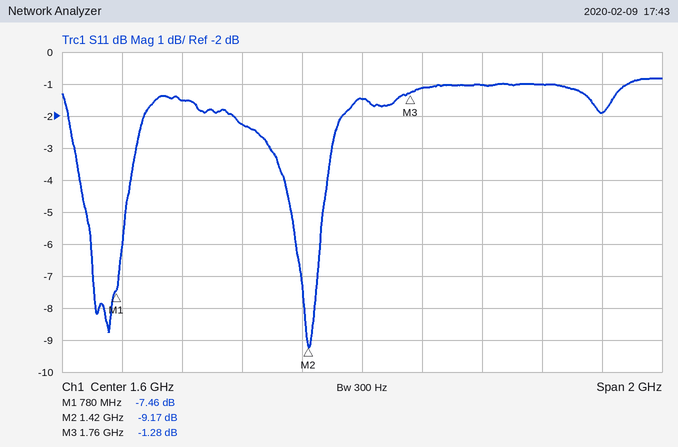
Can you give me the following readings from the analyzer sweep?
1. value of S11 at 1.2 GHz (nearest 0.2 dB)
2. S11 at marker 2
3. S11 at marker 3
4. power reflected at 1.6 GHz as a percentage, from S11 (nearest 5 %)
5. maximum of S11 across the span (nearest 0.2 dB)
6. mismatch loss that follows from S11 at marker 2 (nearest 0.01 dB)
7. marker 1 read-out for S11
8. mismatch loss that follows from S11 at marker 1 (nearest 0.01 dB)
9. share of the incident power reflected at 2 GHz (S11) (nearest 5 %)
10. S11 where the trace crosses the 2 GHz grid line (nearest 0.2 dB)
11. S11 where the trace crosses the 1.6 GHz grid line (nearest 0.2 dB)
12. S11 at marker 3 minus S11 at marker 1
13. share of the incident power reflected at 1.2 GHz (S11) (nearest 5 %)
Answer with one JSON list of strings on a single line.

["-2.2 dB", "-9.17 dB", "-1.28 dB", "70 %", "-0.8 dB", "0.56 dB", "-7.46 dB", "0.86 dB", "80 %", "-1.0 dB", "-1.4 dB", "6.18 dB", "60 %"]
